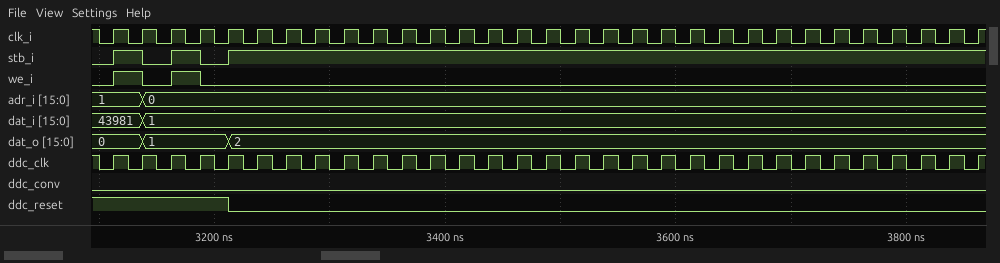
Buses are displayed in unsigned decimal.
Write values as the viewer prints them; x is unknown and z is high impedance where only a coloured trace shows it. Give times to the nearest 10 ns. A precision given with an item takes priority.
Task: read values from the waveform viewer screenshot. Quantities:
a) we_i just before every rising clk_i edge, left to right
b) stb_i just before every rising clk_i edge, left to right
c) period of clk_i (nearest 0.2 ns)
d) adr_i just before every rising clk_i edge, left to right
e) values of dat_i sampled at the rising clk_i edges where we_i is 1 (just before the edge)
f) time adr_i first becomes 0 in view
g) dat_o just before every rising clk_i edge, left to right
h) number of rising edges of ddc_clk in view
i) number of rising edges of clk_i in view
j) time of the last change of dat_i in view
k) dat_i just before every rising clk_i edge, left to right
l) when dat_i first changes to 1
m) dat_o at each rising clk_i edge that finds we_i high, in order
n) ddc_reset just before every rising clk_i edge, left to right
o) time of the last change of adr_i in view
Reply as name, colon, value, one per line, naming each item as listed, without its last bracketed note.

we_i just before every rising clk_i edge, left to right: 0 1 0 1 0 0 0 0 0 0 0 0 0 0 0 0 0 0 0 0 0 0 0 0 0 0 0 0 0 0 0
stb_i just before every rising clk_i edge, left to right: 0 1 0 1 0 1 1 1 1 1 1 1 1 1 1 1 1 1 1 1 1 1 1 1 1 1 1 1 1 1 1
period of clk_i: 25 ns
adr_i just before every rising clk_i edge, left to right: 1, 1, 0, 0, 0, 0, 0, 0, 0, 0, 0, 0, 0, 0, 0, 0, 0, 0, 0, 0, 0, 0, 0, 0, 0, 0, 0, 0, 0, 0, 0
values of dat_i sampled at the rising clk_i edges where we_i is 1: 43981, 1
time adr_i first becomes 0 in view: 3140 ns
dat_o just before every rising clk_i edge, left to right: 0, 0, 1, 1, 1, 2, 2, 2, 2, 2, 2, 2, 2, 2, 2, 2, 2, 2, 2, 2, 2, 2, 2, 2, 2, 2, 2, 2, 2, 2, 2
number of rising edges of ddc_clk in view: 31
number of rising edges of clk_i in view: 31
time of the last change of dat_i in view: 3140 ns
dat_i just before every rising clk_i edge, left to right: 43981, 43981, 1, 1, 1, 1, 1, 1, 1, 1, 1, 1, 1, 1, 1, 1, 1, 1, 1, 1, 1, 1, 1, 1, 1, 1, 1, 1, 1, 1, 1
when dat_i first changes to 1: 3140 ns
dat_o at each rising clk_i edge that finds we_i high, in order: 0, 1
ddc_reset just before every rising clk_i edge, left to right: 1 1 1 1 1 0 0 0 0 0 0 0 0 0 0 0 0 0 0 0 0 0 0 0 0 0 0 0 0 0 0
time of the last change of adr_i in view: 3140 ns
